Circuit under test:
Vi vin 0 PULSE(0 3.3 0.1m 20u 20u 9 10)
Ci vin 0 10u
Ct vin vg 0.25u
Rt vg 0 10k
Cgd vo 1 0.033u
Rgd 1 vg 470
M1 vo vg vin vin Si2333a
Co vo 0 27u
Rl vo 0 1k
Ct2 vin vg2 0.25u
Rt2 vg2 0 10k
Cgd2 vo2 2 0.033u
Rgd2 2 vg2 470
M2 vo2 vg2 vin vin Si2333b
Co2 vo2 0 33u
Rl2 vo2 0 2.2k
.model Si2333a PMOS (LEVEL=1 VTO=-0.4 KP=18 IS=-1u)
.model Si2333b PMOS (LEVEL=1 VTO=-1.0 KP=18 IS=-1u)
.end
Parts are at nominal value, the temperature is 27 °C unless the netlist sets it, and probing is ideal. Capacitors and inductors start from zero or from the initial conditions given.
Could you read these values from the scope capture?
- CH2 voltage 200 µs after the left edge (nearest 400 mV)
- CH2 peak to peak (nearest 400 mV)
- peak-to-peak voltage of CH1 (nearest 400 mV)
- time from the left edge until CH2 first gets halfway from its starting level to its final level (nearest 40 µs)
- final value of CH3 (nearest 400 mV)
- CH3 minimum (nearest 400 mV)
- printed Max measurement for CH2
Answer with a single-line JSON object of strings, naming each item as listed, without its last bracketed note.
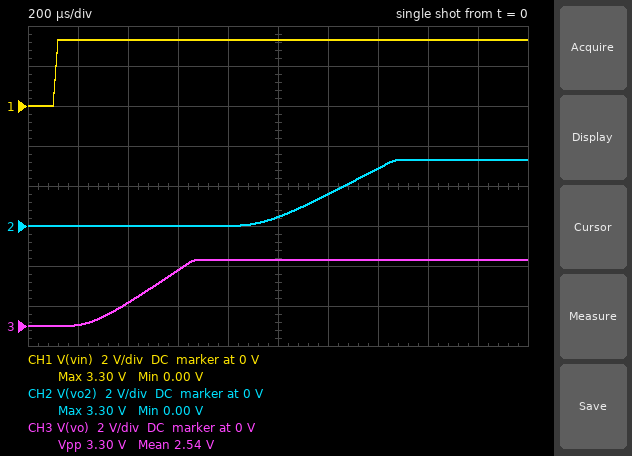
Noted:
{"CH2 voltage 200 µs after the left edge": "0 V", "CH2 peak to peak": "3.2 V", "peak-to-peak voltage of CH1": "3.2 V", "time from the left edge until CH2 first gets halfway from its starting level to its final level": "1.20 ms", "final value of CH3": "3.2 V", "CH3 minimum": "0 V", "printed Max measurement for CH2": "3.30 V"}
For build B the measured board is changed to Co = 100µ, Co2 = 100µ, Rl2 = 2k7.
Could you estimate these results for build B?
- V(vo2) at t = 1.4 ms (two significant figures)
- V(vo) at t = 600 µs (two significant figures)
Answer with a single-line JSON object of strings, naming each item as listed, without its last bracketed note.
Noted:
{"V(vo2) at t = 1.4 ms": "1.9 V", "V(vo) at t = 600 µs": "1.7 V"}
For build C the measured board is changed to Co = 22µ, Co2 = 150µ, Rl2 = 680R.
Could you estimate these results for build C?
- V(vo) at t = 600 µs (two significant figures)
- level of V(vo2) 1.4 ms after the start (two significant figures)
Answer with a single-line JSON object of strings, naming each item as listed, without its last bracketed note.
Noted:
{"V(vo) at t = 600 µs": "2.9 V", "level of V(vo2) 1.4 ms after the start": "1.6 V"}
